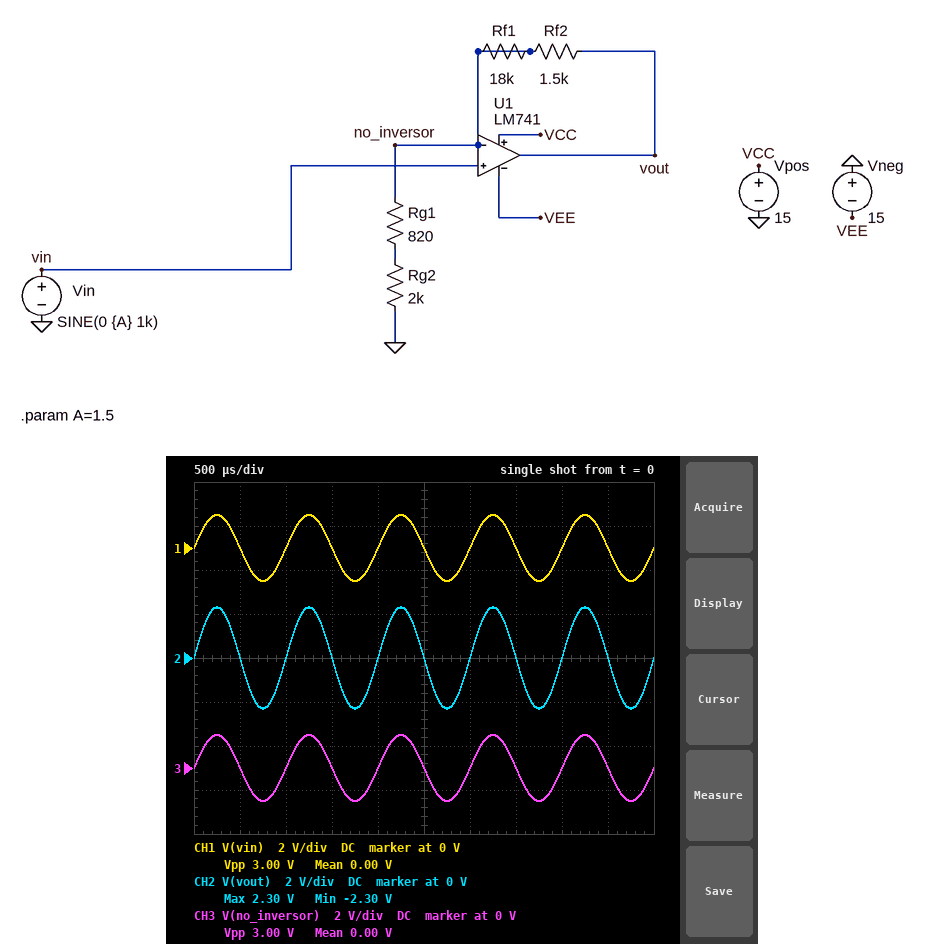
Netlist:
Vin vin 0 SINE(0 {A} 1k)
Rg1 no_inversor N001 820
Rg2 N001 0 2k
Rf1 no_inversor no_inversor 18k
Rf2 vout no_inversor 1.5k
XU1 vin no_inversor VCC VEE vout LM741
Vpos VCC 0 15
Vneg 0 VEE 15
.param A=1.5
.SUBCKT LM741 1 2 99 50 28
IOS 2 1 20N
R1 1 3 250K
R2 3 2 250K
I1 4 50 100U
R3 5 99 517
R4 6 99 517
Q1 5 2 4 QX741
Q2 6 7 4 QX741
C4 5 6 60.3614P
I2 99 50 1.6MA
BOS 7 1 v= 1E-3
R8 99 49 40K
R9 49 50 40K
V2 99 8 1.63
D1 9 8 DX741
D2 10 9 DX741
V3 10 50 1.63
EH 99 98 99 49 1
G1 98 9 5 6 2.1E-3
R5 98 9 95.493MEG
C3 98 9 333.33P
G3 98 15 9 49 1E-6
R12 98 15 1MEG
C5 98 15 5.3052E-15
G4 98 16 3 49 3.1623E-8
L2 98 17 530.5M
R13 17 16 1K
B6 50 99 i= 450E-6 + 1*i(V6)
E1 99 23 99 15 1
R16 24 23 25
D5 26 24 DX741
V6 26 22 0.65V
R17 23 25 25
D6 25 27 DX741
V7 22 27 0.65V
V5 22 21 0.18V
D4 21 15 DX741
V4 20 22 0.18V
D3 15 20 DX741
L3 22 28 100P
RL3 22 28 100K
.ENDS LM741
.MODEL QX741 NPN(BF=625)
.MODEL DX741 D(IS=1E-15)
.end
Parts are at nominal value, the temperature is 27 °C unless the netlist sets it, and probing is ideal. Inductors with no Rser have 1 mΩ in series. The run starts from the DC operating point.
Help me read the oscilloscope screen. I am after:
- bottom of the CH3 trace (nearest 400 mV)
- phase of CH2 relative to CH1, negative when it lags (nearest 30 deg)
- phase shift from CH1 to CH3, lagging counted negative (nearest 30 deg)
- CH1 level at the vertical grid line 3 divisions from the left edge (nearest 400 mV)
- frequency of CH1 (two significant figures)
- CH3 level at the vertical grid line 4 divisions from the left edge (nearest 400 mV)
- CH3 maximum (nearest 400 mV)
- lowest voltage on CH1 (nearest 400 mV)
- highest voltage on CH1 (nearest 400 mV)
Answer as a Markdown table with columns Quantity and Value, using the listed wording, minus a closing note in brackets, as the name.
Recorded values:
| Quantity | Value |
|---|---|
| bottom of the CH3 trace | -1.6 V |
| phase of CH2 relative to CH1, negative when it lags | 0 deg |
| phase shift from CH1 to CH3, lagging counted negative | 0 deg |
| CH1 level at the vertical grid line 3 divisions from the left edge | 0 V |
| frequency of CH1 | 1.0 kHz |
| CH3 level at the vertical grid line 4 divisions from the left edge | 0 V |
| CH3 maximum | 1.6 V |
| lowest voltage on CH1 | -1.6 V |
| highest voltage on CH1 | 1.6 V |
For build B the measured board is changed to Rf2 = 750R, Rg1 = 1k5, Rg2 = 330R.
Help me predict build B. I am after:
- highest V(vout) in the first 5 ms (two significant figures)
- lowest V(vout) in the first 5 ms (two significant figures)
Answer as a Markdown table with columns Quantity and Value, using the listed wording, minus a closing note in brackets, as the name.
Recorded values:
| Quantity | Value |
|---|---|
| highest V(vout) in the first 5 ms | 2.1 V |
| lowest V(vout) in the first 5 ms | -2.1 V |
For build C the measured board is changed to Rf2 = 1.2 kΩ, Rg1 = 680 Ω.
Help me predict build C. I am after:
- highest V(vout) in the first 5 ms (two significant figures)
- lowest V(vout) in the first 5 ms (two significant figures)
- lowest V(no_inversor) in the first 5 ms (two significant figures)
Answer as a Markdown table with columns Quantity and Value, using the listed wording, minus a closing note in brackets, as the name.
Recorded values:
| Quantity | Value |
|---|---|
| highest V(vout) in the first 5 ms | 2.2 V |
| lowest V(vout) in the first 5 ms | -2.2 V |
| lowest V(no_inversor) in the first 5 ms | -1.5 V |
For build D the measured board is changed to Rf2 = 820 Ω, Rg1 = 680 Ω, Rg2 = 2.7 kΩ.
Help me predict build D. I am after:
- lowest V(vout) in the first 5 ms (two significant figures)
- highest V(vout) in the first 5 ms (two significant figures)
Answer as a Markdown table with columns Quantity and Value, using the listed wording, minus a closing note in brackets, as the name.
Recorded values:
| Quantity | Value |
|---|---|
| lowest V(vout) in the first 5 ms | -1.9 V |
| highest V(vout) in the first 5 ms | 1.9 V |
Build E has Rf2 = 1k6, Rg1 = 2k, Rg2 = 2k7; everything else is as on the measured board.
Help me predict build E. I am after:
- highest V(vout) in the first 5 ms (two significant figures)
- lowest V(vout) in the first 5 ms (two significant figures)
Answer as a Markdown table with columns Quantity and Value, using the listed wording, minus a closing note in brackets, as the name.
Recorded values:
| Quantity | Value |
|---|---|
| highest V(vout) in the first 5 ms | 2.0 V |
| lowest V(vout) in the first 5 ms | -2.0 V |
